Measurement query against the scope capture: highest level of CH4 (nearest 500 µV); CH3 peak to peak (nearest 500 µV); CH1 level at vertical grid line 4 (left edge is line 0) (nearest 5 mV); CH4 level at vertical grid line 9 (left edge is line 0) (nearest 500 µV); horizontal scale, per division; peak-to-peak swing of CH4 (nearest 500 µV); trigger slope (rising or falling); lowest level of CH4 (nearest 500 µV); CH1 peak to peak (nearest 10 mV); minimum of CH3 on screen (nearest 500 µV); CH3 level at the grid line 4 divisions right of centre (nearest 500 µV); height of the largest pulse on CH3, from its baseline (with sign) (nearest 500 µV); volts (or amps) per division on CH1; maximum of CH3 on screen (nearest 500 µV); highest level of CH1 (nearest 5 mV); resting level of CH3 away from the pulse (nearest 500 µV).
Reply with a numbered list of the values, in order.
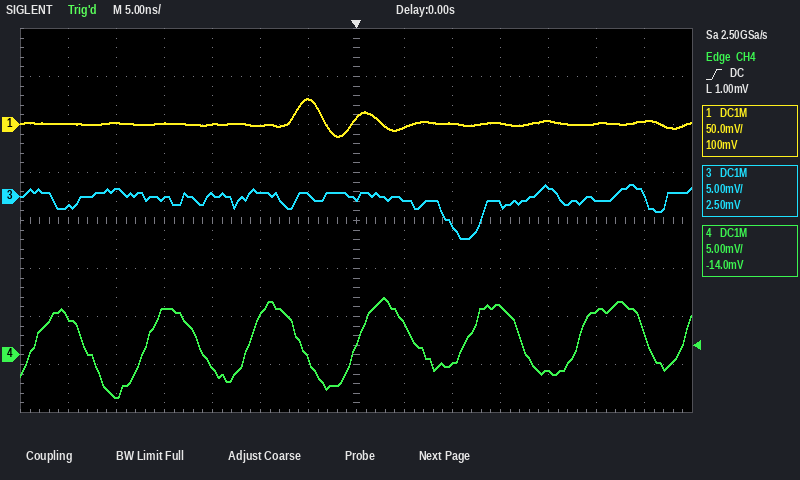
1. 6.0 mV
2. 5.5 mV
3. 0 mV
4. -1.0 mV
5. 5 ns
6. 10.5 mV
7. rising
8. -4.5 mV
9. 40 mV
10. -4.5 mV
11. 1.0 mV
12. -4.5 mV
13. 50 mV
14. 1.0 mV
15. 25 mV
16. 0.0 mV
